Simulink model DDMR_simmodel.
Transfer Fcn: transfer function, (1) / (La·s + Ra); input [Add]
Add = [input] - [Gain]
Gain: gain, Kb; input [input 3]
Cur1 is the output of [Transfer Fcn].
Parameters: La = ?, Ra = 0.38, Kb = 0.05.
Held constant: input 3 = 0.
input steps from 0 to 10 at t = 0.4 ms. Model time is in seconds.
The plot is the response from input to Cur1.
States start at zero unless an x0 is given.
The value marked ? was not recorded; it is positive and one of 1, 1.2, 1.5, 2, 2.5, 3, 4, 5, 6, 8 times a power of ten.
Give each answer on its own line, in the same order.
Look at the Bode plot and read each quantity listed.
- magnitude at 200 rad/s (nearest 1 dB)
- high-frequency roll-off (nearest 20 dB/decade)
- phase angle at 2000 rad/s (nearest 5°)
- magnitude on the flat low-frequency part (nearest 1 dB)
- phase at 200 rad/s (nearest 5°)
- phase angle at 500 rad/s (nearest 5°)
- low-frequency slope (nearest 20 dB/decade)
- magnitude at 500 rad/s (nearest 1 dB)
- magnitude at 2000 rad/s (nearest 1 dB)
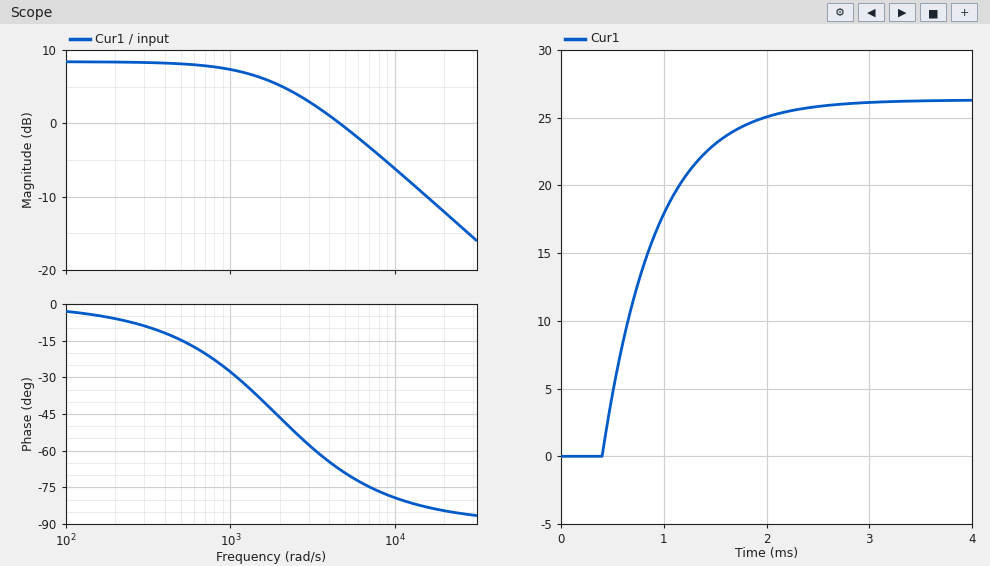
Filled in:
8 dB
-20 dB/decade
-45°
8 dB
-5°
-15°
0 dB/decade
8 dB
5 dB
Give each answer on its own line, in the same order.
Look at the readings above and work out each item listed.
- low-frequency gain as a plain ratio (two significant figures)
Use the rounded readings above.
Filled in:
2.5
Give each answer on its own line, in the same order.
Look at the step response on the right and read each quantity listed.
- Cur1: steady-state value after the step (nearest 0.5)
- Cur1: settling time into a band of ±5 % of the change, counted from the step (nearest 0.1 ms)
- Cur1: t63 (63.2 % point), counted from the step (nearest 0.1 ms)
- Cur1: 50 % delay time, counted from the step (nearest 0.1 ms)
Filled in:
26.5
1.6 ms
0.5 ms
0.4 ms
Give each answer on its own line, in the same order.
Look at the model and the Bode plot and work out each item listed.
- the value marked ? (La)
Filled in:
0.0002
